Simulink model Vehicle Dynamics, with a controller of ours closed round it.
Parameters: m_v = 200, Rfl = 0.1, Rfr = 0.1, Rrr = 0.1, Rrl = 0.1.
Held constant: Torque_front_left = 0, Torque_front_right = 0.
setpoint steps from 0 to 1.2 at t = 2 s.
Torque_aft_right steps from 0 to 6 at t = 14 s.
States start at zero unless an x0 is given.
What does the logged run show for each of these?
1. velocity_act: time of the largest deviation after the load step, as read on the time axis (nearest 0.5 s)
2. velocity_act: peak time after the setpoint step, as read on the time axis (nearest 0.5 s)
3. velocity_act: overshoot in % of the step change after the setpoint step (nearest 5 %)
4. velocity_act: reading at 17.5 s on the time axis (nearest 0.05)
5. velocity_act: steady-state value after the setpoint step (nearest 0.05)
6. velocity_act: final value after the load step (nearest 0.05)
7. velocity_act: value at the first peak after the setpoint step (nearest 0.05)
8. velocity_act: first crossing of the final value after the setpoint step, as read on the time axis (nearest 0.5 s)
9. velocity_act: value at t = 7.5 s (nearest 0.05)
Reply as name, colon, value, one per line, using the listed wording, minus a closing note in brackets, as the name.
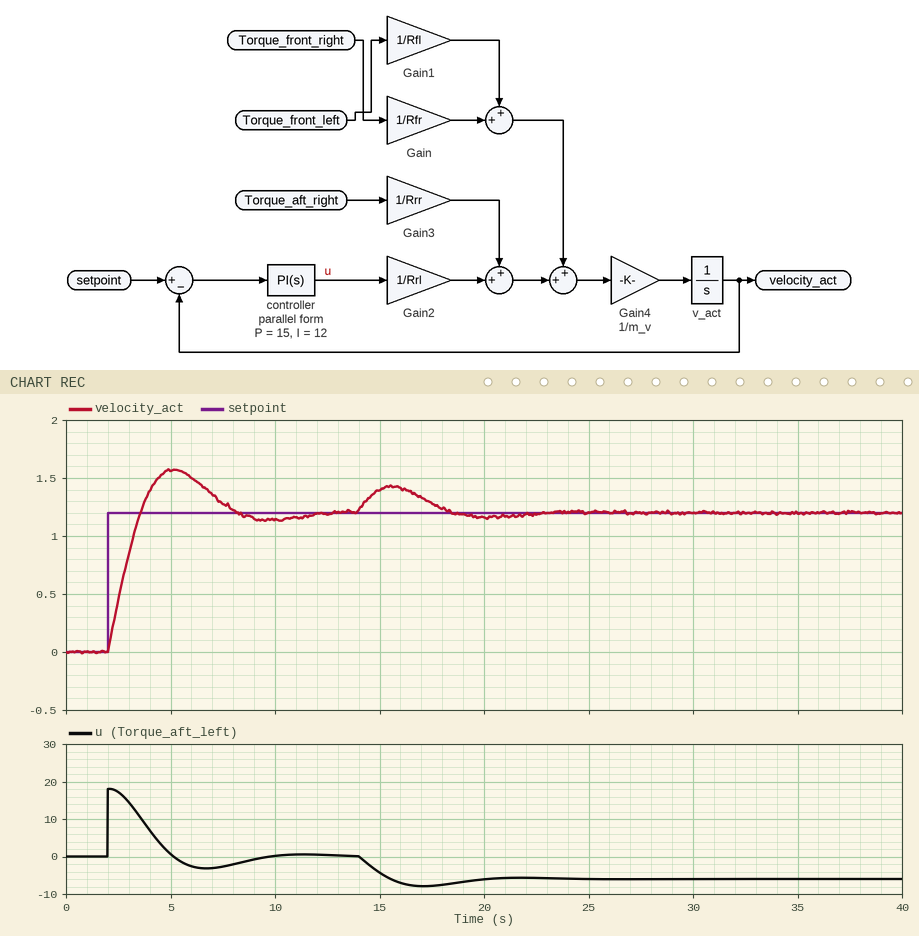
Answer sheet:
velocity_act: time of the largest deviation after the load step, as read on the time axis: 15.5 s
velocity_act: peak time after the setpoint step, as read on the time axis: 5.0 s
velocity_act: overshoot in % of the step change after the setpoint step: 30 %
velocity_act: reading at 17.5 s on the time axis: 1.30
velocity_act: steady-state value after the setpoint step: 1.20
velocity_act: final value after the load step: 1.20
velocity_act: value at the first peak after the setpoint step: 1.55
velocity_act: first crossing of the final value after the setpoint step, as read on the time axis: 3.5 s
velocity_act: value at t = 7.5 s: 1.30
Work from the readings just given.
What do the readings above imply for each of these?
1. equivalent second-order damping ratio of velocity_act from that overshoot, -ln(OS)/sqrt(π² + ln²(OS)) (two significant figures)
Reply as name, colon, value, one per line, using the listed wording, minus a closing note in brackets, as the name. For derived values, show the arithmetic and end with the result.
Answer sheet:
equivalent second-order damping ratio of velocity_act from that overshoot, -ln(OS)/sqrt(π² + ln²(OS)): ln(0.3) = -1.204; 1.204 / sqrt(9.870 + 1.450) = 0.36
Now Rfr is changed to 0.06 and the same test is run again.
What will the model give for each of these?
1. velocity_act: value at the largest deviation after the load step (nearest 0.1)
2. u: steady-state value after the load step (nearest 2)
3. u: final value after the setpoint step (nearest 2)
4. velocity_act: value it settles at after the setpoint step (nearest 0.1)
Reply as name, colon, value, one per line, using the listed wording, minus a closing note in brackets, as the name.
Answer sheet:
velocity_act: value at the largest deviation after the load step: 1.4
u: steady-state value after the load step: -6
u: final value after the setpoint step: 0
velocity_act: value it settles at after the setpoint step: 1.2
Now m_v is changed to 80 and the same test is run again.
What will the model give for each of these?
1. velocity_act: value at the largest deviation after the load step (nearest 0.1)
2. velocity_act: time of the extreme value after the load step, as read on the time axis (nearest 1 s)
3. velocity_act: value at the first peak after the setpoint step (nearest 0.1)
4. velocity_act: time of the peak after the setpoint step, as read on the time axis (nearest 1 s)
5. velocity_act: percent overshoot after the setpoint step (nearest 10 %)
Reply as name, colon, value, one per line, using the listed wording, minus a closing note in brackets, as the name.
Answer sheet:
velocity_act: value at the largest deviation after the load step: 1.5
velocity_act: time of the extreme value after the load step, as read on the time axis: 15 s
velocity_act: value at the first peak after the setpoint step: 1.4
velocity_act: time of the peak after the setpoint step, as read on the time axis: 4 s
velocity_act: percent overshoot after the setpoint step: 20 %
